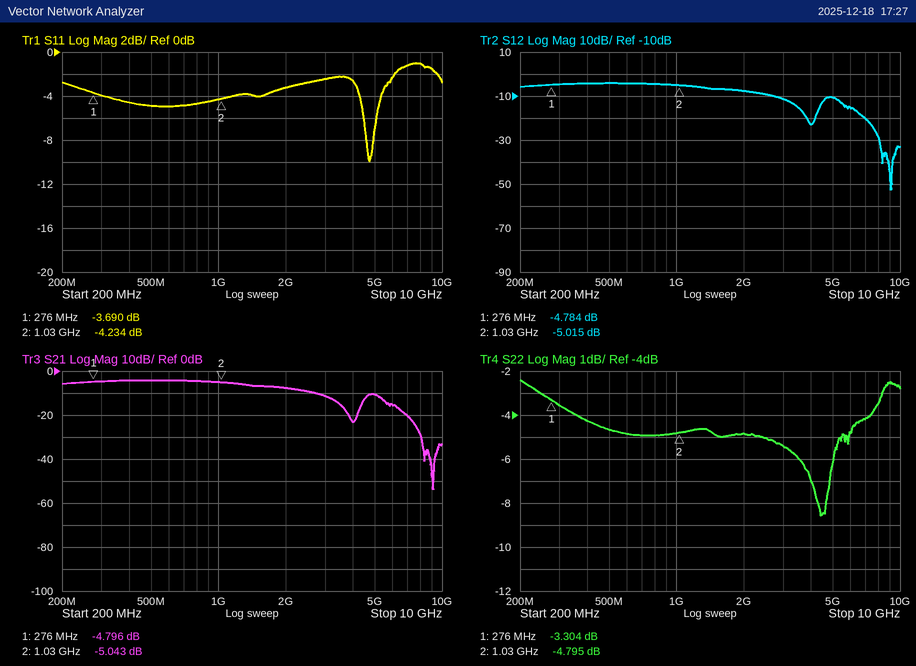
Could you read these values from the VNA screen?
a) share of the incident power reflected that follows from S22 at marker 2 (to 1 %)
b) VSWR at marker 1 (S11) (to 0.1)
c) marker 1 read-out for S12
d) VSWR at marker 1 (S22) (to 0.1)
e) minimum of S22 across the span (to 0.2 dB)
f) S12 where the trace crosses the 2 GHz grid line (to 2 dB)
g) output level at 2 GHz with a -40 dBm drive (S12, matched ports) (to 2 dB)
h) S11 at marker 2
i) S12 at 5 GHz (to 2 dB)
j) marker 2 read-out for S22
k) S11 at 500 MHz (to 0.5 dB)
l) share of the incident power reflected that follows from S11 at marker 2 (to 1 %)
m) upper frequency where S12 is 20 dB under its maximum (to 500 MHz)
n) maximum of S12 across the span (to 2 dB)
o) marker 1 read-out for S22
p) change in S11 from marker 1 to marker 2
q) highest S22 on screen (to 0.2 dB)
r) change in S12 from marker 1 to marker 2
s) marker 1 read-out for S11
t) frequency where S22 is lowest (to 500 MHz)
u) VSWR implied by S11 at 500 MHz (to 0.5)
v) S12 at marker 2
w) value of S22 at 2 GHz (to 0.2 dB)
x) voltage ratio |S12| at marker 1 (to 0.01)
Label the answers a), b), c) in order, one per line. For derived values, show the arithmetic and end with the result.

a) 10^(-4.795/10) ≈ 33 %
b) (1 + 0.6539)/(1 − 0.6539) ≈ 4.8
c) -4.784 dB
d) (1 + 0.6836)/(1 − 0.6836) ≈ 5.3
e) -8.6 dB
f) -8 dB
g) -40 dBm + (-8 dB) = -48 dBm
h) -4.234 dB
i) -10 dB
j) -4.795 dB
k) -5.0 dB
l) 10^(-4.234/10) ≈ 38 %
m) 7.5 GHz
n) -4 dB
o) -3.304 dB
p) -4.234 − (-3.69) = -0.544 dB
q) -2.4 dB
r) -5.015 − (-4.784) = -0.231 dB
s) -3.690 dB
t) 4.5 GHz
u) |Γ| = 10^(-5/20) = 0.5623; VSWR = (1 + 0.5623)/(1 − 0.5623) ≈ 3.57, so 3.5 to the nearest 0.5
v) -5.015 dB
w) -4.8 dB
x) 10^(-4.784/20) ≈ 0.58
